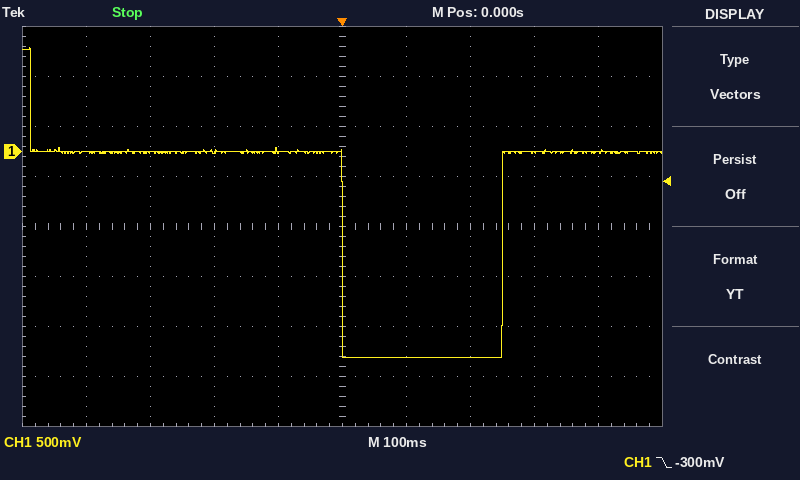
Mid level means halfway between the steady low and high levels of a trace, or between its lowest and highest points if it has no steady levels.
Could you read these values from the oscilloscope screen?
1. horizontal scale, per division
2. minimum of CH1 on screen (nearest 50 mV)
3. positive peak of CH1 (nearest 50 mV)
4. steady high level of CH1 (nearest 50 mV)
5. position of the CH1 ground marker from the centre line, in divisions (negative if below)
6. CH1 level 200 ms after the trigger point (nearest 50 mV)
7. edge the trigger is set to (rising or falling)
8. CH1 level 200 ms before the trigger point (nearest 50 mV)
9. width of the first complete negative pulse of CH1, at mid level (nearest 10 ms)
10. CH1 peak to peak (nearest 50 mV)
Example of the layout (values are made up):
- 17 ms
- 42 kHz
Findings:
- 100 ms
- -2.05 V
- 1.05 V
- 0 mV
- +1.5 div
- -2.05 V
- falling
- 0 mV
- 250 ms
- 3.10 V
